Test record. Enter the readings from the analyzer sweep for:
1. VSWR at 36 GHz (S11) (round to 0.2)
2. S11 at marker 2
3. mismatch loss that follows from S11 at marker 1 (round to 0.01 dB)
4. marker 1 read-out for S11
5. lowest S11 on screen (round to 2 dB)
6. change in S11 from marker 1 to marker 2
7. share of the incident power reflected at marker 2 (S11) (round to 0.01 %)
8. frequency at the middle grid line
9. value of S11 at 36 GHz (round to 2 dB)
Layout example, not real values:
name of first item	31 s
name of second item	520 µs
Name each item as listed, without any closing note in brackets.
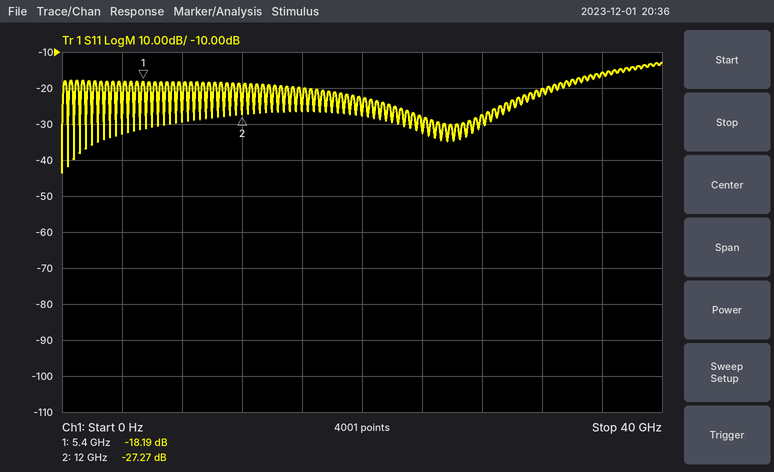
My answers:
VSWR at 36 GHz (S11)	1.4
S11 at marker 2	-27.27 dB
mismatch loss that follows from S11 at marker 1	0.07 dB
marker 1 read-out for S11	-18.19 dB
lowest S11 on screen	-44 dB
change in S11 from marker 1 to marker 2	-9.08 dB
share of the incident power reflected at marker 2 (S11)	0.19 %
frequency at the middle grid line	20 GHz
value of S11 at 36 GHz	-16 dB
